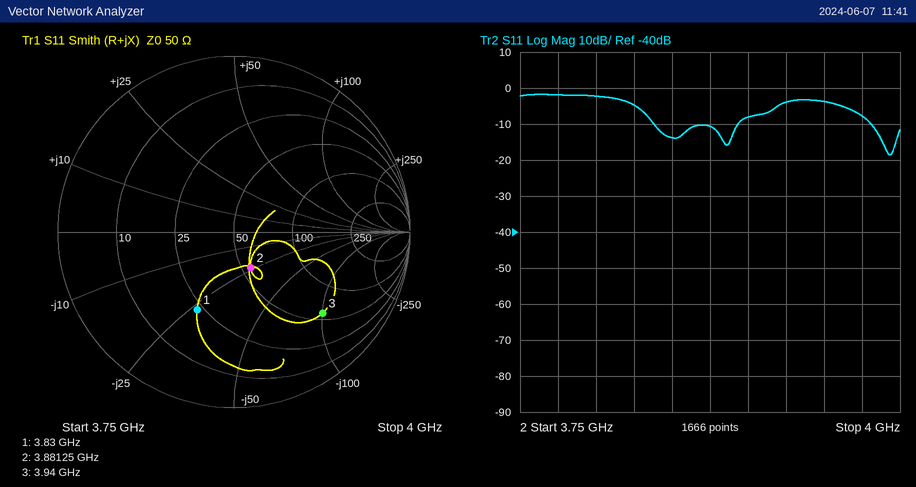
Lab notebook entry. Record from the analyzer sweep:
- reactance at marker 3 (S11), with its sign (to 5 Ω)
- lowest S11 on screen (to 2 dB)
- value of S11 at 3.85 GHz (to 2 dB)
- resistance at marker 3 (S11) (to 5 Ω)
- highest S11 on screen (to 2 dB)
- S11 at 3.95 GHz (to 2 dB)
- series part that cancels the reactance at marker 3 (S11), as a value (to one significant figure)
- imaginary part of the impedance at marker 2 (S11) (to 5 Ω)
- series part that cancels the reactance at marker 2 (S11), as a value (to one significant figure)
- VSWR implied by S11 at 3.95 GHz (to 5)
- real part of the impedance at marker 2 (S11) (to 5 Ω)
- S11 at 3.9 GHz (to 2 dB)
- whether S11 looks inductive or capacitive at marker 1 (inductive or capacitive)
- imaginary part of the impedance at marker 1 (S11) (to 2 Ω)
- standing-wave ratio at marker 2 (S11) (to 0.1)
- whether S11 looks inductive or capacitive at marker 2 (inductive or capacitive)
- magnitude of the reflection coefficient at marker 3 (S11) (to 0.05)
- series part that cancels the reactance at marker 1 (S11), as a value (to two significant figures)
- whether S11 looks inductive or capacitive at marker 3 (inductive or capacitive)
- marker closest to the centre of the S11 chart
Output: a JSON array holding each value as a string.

["-100 Ω", "-18 dB", "-14 dB", "60 Ω", "-2 dB", "-4 dB", "4 nH", "-25 Ω", "1.0 nH", "5", "55 Ω", "-8 dB", "capacitive", "-26 Ω", "1.6", "capacitive", "0.70", "1.1 nH", "capacitive", "marker 2"]
